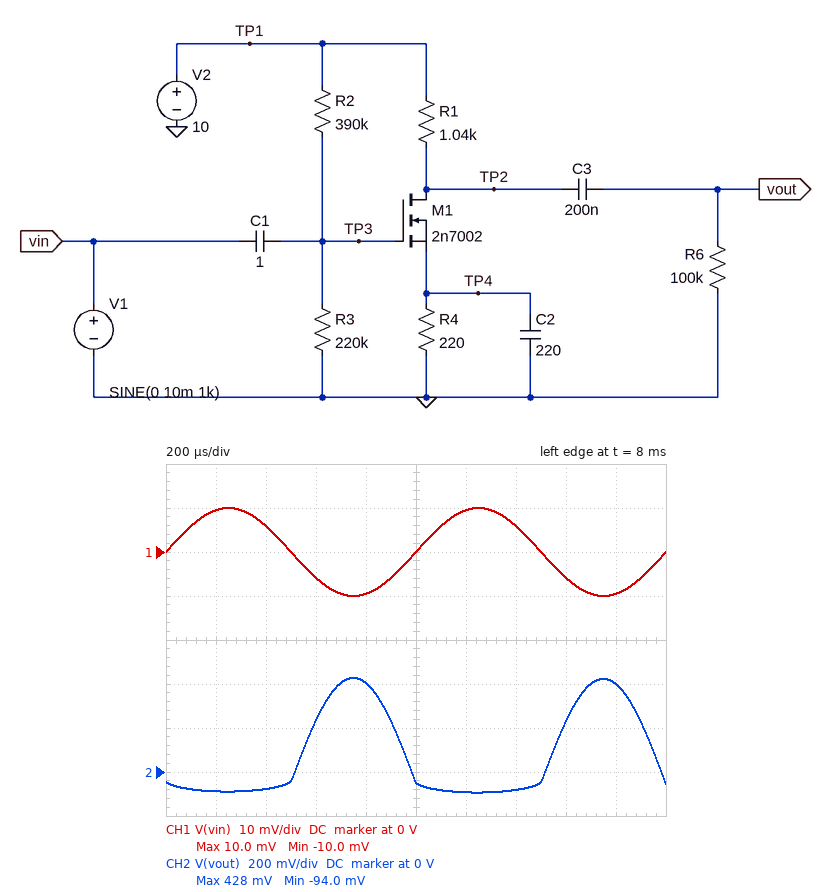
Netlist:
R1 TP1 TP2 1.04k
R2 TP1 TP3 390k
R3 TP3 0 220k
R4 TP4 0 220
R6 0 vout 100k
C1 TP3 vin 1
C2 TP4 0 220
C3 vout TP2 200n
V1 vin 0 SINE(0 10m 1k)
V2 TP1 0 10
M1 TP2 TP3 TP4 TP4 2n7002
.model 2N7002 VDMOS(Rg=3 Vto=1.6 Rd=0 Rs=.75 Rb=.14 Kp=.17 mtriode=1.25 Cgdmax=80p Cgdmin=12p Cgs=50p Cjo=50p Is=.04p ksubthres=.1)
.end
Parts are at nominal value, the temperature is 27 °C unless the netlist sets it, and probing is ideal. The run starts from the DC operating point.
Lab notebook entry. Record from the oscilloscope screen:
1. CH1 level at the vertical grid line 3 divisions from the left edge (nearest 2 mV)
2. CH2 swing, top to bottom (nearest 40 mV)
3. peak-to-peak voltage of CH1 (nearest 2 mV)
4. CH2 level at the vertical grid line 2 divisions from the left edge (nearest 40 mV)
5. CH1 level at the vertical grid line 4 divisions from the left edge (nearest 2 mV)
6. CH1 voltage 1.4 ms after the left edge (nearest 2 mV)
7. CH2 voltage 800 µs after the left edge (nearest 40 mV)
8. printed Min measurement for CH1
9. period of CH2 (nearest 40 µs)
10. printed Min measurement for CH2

-6 mV
520 mV
20 mV
-80 mV
-10 mV
6 mV
400 mV
-10.0 mV
1.00 ms
-94.0 mV
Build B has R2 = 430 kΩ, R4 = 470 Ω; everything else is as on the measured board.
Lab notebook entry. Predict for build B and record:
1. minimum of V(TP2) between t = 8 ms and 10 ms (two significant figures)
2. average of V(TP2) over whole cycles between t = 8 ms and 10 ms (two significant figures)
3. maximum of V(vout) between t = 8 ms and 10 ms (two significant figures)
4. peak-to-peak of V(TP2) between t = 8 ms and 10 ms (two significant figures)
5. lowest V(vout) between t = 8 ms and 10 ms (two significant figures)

6.2 V
6.5 V
290 mV
590 mV
-300 mV
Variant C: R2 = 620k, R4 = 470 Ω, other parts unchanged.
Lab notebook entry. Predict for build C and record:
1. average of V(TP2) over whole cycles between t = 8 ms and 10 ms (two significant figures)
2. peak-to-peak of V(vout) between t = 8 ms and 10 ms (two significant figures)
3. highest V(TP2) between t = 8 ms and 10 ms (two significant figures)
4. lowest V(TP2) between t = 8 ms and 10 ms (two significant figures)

8.0 V
400 mV
8.2 V
7.8 V
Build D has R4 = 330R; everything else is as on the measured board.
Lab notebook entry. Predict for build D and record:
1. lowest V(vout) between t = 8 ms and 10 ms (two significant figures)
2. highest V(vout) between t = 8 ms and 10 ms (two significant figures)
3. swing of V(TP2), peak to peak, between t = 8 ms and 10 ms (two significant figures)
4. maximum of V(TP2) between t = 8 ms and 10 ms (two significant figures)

-400 mV
390 mV
780 mV
4.8 V
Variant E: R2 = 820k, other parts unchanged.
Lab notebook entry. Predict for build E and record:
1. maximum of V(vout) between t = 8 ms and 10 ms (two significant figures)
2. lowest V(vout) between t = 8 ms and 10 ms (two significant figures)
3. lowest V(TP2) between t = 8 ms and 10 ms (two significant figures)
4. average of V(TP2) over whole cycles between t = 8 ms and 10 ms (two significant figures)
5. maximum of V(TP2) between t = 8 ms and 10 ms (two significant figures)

190 mV
-200 mV
7.9 V
8.1 V
8.3 V
